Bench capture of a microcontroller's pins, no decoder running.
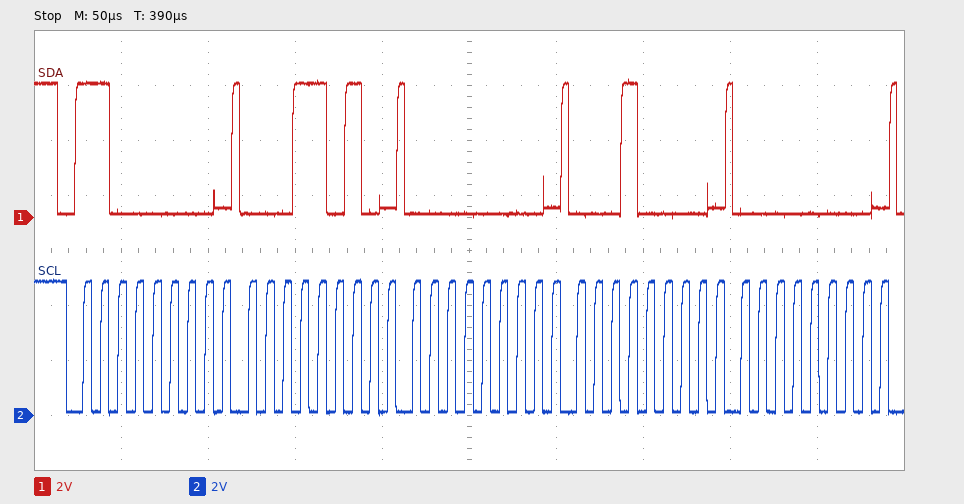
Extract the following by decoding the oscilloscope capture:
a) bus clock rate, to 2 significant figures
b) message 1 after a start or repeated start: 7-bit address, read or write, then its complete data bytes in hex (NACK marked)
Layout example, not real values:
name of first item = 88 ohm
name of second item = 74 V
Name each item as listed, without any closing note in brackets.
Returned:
bus clock rate, to 2 significant figures = 100 kHz
message 1 after a start or repeated start: 7-bit address, read or write, then its complete data bytes in hex = 0x60 write: 1A 00 10 00
